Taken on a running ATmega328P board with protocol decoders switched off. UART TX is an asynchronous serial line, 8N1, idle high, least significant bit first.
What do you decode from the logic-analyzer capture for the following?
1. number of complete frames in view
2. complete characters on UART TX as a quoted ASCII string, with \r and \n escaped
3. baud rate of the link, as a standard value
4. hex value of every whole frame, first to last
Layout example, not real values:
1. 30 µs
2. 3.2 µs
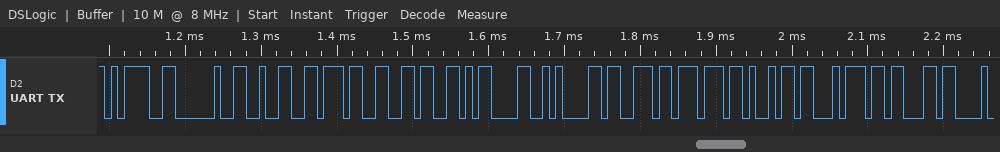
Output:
1. 12
2. "= 276\r\nswitc"
3. 115200 baud
4. 3D 20 32 37 36 0D 0A 73 77 69 74 63
